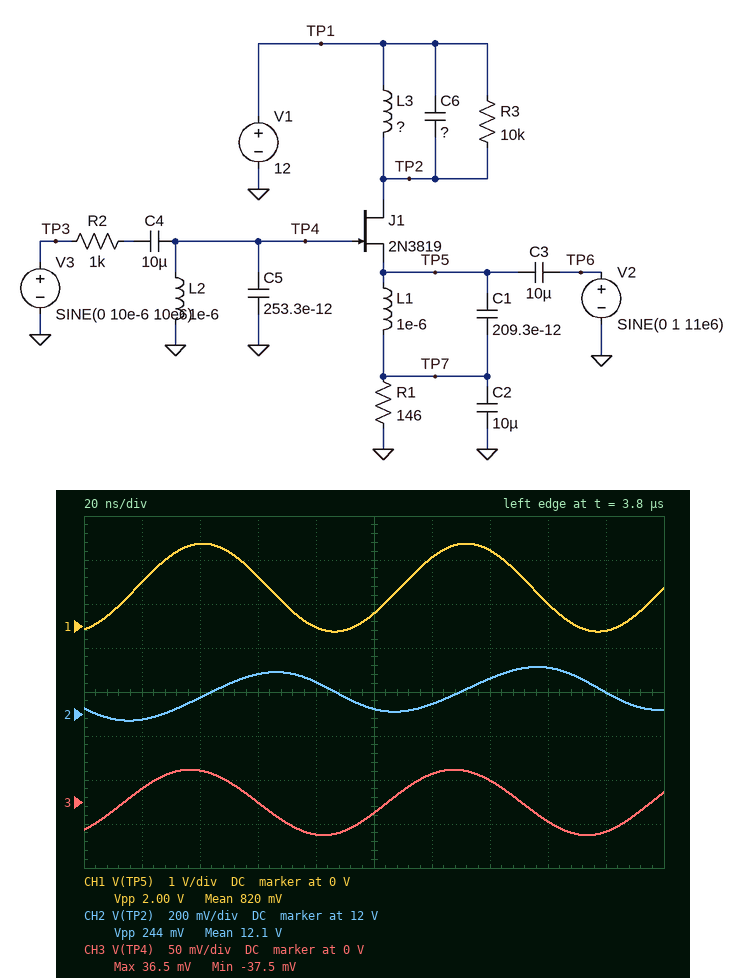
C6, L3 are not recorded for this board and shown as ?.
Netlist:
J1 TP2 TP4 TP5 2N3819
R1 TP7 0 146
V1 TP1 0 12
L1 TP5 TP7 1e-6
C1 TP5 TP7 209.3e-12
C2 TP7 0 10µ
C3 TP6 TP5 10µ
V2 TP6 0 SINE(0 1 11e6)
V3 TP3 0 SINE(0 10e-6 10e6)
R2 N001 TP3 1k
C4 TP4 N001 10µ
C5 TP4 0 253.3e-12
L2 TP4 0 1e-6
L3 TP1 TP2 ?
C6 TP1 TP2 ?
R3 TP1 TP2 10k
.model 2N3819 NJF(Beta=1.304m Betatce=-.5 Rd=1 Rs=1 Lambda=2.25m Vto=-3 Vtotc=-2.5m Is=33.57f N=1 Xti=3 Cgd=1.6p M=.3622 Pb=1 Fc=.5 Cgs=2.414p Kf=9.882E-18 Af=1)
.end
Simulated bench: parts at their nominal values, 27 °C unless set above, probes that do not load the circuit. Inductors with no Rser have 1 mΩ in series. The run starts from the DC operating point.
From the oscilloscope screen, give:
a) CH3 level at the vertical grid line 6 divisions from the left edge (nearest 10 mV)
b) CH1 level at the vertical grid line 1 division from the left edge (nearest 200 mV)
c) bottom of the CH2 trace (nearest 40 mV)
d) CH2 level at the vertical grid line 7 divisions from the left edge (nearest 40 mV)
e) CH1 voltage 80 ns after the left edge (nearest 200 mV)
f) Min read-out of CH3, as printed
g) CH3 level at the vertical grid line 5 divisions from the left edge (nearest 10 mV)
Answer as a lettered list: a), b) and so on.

a) 30 mV
b) 1.0 V
c) 11.96 V
d) 12.16 V
e) 0 V
f) -37.5 mV
g) -10 mV
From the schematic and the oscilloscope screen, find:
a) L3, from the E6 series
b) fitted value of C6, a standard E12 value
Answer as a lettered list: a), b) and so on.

a) 33 µH
b) 820 pF
